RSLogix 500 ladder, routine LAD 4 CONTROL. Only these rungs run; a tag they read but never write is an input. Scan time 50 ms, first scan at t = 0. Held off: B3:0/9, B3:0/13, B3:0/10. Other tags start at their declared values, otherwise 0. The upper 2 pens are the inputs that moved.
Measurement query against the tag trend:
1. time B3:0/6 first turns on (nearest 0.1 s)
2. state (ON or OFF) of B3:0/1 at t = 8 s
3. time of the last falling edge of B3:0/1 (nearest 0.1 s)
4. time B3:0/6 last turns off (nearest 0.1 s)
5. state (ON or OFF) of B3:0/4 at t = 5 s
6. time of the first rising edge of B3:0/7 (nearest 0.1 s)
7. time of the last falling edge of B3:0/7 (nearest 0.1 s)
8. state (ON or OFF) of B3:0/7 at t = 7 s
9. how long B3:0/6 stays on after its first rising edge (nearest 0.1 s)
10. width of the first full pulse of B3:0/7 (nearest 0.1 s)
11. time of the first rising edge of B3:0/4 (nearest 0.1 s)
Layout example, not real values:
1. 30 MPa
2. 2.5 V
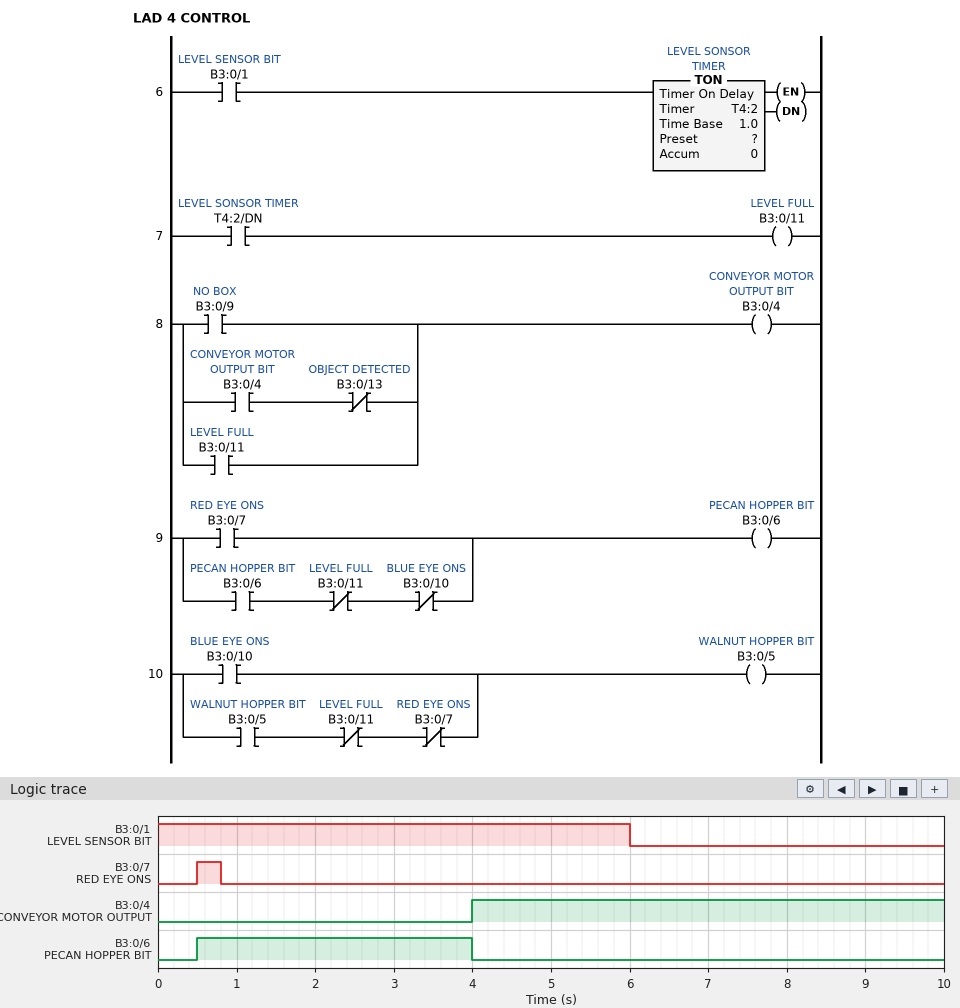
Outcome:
1. 0.5 s
2. OFF
3. 6.0 s
4. 4.0 s
5. ON
6. 0.5 s
7. 0.8 s
8. OFF
9. 3.5 s
10. 0.3 s
11. 4.0 s
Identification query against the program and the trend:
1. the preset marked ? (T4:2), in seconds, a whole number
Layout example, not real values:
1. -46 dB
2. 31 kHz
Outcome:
1. 4 s
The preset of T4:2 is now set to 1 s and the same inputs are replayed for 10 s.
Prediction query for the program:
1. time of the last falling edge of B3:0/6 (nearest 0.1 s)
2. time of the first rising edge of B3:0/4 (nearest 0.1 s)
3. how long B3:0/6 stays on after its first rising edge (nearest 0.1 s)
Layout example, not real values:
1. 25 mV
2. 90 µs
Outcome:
1. 1.0 s
2. 1.0 s
3. 0.5 s
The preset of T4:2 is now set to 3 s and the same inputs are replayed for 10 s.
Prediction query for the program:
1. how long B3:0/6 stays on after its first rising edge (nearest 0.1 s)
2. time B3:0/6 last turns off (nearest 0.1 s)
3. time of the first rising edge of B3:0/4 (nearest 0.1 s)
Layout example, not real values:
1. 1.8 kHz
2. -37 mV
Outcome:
1. 2.5 s
2. 3.0 s
3. 3.0 s
